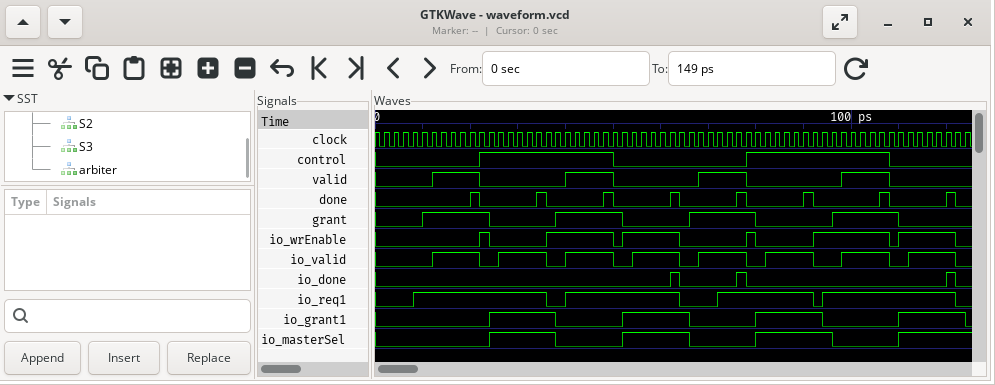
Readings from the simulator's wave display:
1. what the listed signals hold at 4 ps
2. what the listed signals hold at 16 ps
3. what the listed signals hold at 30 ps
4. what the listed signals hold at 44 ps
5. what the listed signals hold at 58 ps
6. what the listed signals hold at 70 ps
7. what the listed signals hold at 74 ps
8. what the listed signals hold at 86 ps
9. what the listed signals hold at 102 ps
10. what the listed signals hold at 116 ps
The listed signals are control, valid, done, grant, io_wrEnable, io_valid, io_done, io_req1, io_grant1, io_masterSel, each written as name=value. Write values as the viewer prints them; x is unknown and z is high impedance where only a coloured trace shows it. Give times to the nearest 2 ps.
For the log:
control=0, valid=0, done=0, grant=0, io_wrEnable=0, io_valid=0, io_done=0, io_req1=0, io_grant1=0, io_masterSel=0
control=0, valid=1, done=0, grant=1, io_wrEnable=0, io_valid=1, io_done=0, io_req1=1, io_grant1=0, io_masterSel=0
control=1, valid=0, done=0, grant=0, io_wrEnable=0, io_valid=1, io_done=0, io_req1=1, io_grant1=1, io_masterSel=1
control=1, valid=1, done=0, grant=1, io_wrEnable=1, io_valid=1, io_done=0, io_req1=1, io_grant1=0, io_masterSel=0
control=0, valid=0, done=0, grant=0, io_wrEnable=1, io_valid=1, io_done=0, io_req1=1, io_grant1=1, io_masterSel=1
control=0, valid=1, done=0, grant=1, io_wrEnable=0, io_valid=1, io_done=0, io_req1=0, io_grant1=0, io_masterSel=0
control=0, valid=1, done=0, grant=1, io_wrEnable=0, io_valid=1, io_done=0, io_req1=1, io_grant1=0, io_masterSel=0
control=1, valid=0, done=0, grant=0, io_wrEnable=0, io_valid=1, io_done=0, io_req1=1, io_grant1=1, io_masterSel=1
control=1, valid=1, done=0, grant=1, io_wrEnable=1, io_valid=1, io_done=0, io_req1=1, io_grant1=0, io_masterSel=0
control=0, valid=0, done=0, grant=0, io_wrEnable=1, io_valid=1, io_done=0, io_req1=1, io_grant1=1, io_masterSel=1
